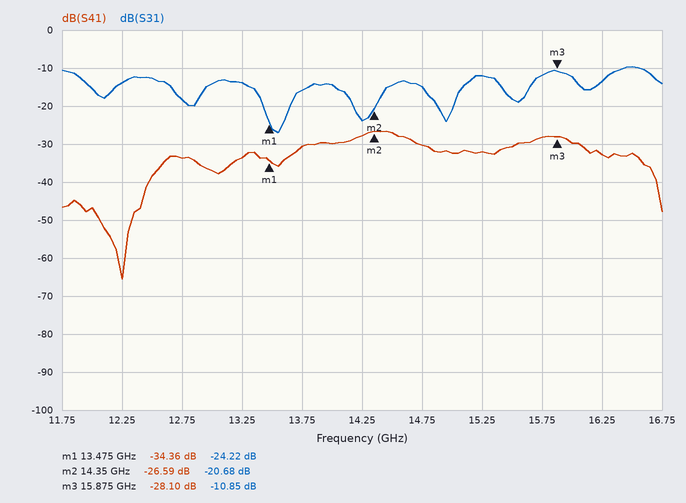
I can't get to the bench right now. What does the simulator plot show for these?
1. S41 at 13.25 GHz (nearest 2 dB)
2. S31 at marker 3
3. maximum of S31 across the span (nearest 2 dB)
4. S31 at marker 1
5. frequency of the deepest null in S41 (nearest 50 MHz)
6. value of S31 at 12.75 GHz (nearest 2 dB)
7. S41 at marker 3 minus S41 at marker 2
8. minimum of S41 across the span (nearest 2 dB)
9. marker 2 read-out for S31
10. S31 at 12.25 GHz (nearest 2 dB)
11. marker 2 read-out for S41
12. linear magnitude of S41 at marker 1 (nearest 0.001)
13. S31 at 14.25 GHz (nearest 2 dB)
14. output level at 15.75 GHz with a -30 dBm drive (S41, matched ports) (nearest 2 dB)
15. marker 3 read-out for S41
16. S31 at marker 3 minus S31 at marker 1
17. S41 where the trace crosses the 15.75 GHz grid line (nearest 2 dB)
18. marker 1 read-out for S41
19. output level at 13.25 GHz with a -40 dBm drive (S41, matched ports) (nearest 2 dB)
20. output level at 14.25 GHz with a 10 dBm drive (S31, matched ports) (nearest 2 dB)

-34 dB
-10.85 dB
-10 dB
-24.22 dB
12.25 GHz
-18 dB
-1.51 dB
-66 dB
-20.68 dB
-14 dB
-26.59 dB
0.019
-24 dB
-58 dBm
-28.10 dB
13.37 dB
-28 dB
-34.36 dB
-74 dBm
-14 dBm
